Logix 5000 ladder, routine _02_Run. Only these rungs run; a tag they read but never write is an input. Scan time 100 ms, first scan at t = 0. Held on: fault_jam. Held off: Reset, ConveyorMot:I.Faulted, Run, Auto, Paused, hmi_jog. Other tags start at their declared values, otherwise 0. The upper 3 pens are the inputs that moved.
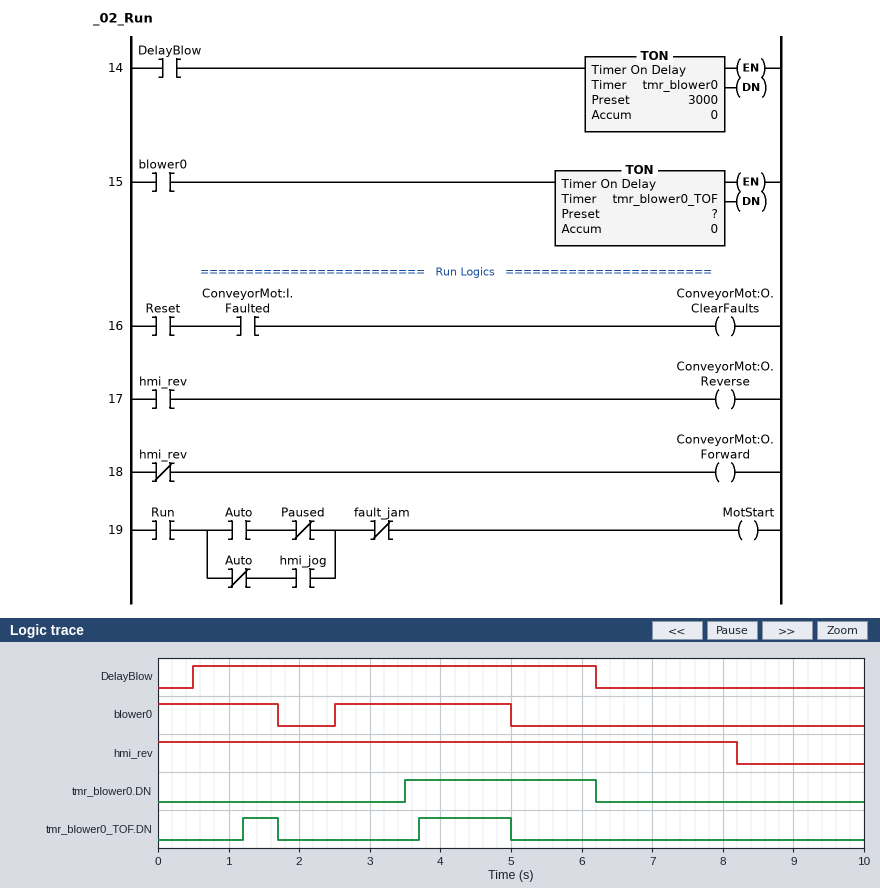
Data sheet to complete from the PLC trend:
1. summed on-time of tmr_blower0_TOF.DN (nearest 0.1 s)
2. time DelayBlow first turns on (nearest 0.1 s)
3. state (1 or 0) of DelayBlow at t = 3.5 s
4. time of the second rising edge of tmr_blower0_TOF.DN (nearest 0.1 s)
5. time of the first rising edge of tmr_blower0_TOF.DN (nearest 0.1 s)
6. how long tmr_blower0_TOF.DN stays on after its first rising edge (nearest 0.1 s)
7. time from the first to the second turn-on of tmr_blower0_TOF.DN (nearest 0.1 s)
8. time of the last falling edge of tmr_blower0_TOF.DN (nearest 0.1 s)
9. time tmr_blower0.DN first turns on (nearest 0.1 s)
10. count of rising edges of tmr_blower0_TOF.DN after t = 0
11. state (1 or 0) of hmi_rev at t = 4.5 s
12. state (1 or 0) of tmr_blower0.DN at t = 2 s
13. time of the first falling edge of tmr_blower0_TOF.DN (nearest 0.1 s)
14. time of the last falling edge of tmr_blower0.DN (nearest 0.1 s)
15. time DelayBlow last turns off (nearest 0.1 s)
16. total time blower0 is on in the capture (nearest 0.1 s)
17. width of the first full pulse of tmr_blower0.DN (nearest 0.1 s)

1.8 s
0.5 s
1
3.7 s
1.2 s
0.5 s
2.5 s
5.0 s
3.5 s
2
1
0
1.7 s
6.2 s
6.2 s
4.2 s
2.7 s
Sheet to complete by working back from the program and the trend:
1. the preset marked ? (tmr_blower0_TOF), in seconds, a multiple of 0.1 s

1.2 s
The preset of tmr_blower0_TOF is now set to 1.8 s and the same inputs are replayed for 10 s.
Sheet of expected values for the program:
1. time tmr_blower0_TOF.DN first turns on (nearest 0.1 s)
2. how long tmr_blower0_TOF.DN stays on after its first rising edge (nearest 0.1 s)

4.3 s
0.7 s
